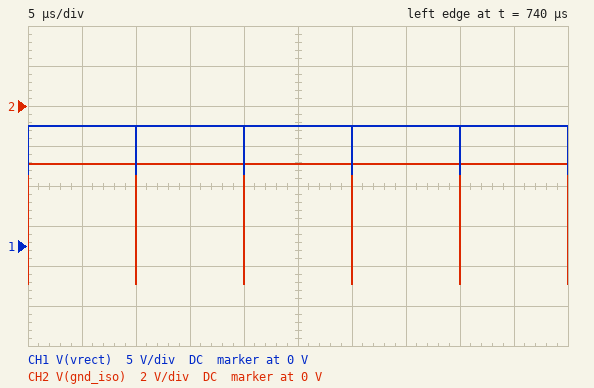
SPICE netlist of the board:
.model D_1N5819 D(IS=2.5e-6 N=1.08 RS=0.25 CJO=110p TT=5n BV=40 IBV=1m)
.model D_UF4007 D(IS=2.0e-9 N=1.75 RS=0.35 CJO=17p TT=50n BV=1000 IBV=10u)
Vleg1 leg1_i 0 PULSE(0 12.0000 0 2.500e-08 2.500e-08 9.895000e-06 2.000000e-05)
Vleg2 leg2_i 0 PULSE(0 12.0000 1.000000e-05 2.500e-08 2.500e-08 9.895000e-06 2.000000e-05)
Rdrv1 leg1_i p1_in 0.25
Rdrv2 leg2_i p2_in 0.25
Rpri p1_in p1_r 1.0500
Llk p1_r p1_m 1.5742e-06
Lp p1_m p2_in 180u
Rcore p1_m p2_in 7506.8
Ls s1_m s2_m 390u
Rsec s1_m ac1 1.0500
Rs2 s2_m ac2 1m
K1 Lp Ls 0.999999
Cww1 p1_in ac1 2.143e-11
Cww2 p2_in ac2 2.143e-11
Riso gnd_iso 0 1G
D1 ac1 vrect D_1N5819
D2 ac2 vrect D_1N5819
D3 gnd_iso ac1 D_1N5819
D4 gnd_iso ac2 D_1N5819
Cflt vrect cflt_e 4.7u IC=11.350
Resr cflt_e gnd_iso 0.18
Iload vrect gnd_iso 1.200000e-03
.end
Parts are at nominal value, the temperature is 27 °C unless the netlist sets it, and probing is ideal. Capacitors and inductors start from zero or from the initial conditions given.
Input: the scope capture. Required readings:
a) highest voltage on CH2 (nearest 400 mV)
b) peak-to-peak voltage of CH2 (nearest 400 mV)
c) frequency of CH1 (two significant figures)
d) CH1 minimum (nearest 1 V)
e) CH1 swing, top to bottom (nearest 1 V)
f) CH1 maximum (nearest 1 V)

-2.8 V
6.0 V
100 kHz
9 V
6 V
15 V
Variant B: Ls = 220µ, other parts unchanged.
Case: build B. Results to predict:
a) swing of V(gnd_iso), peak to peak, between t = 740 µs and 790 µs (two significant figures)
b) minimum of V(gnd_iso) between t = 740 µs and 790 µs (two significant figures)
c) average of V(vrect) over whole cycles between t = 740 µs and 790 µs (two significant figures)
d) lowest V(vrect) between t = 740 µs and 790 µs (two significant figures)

6.0 V
-6.6 V
13 V
6.6 V
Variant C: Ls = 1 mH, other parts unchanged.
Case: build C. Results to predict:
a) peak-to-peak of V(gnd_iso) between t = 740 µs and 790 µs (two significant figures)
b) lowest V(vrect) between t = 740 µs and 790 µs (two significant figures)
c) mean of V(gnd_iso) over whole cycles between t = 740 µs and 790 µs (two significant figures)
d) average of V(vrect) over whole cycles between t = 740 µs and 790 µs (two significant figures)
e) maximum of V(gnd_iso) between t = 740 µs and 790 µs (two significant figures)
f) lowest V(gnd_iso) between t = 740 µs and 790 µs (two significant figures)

6.0 V
14 V
-8.2 V
20 V
-8.1 V
-14 V
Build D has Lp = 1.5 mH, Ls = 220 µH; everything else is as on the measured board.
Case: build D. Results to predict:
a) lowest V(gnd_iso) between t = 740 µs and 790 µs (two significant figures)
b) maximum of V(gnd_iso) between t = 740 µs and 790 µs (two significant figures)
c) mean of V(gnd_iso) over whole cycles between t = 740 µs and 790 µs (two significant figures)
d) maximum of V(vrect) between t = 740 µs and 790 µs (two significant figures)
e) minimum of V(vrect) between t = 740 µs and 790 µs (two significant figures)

-5.6 V
420 mV
370 mV
12 V
5.6 V
